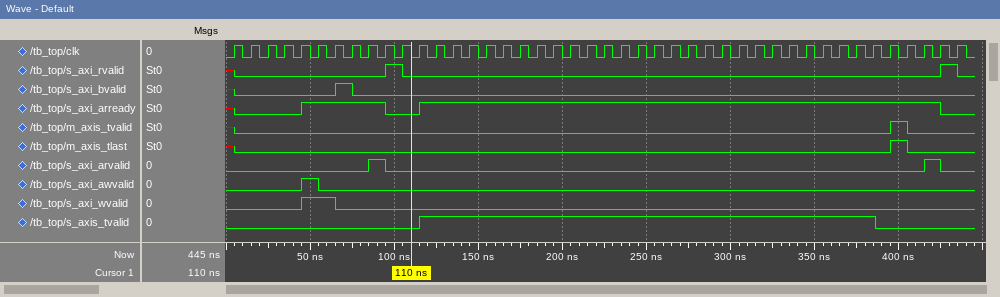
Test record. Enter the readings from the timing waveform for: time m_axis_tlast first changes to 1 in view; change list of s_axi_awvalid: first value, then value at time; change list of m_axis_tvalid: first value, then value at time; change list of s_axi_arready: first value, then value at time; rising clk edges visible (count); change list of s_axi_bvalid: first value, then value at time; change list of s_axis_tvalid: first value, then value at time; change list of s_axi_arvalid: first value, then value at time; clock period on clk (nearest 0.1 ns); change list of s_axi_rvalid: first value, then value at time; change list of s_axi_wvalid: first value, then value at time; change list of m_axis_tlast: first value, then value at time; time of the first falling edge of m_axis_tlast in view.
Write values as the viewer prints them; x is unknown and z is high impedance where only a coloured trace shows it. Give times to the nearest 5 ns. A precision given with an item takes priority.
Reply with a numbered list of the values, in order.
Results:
1. 395 ns
2. 0, 1 at 45 ns, 0 at 55 ns
3. x, 0 at 5 ns, 1 at 395 ns, 0 at 405 ns
4. x, 0 at 5 ns, 1 at 45 ns, 0 at 95 ns, 1 at 115 ns, 0 at 425 ns
5. 44
6. x, 0 at 5 ns, 1 at 65 ns, 0 at 75 ns
7. 0, 1 at 115 ns, 0 at 385 ns
8. 0, 1 at 85 ns, 0 at 95 ns, 1 at 415 ns, 0 at 425 ns
9. 10 ns
10. x, 0 at 5 ns, 1 at 95 ns, 0 at 105 ns, 1 at 425 ns, 0 at 435 ns
11. 0, 1 at 45 ns, 0 at 65 ns
12. x, 0 at 5 ns, 1 at 395 ns, 0 at 405 ns
13. 405 ns
